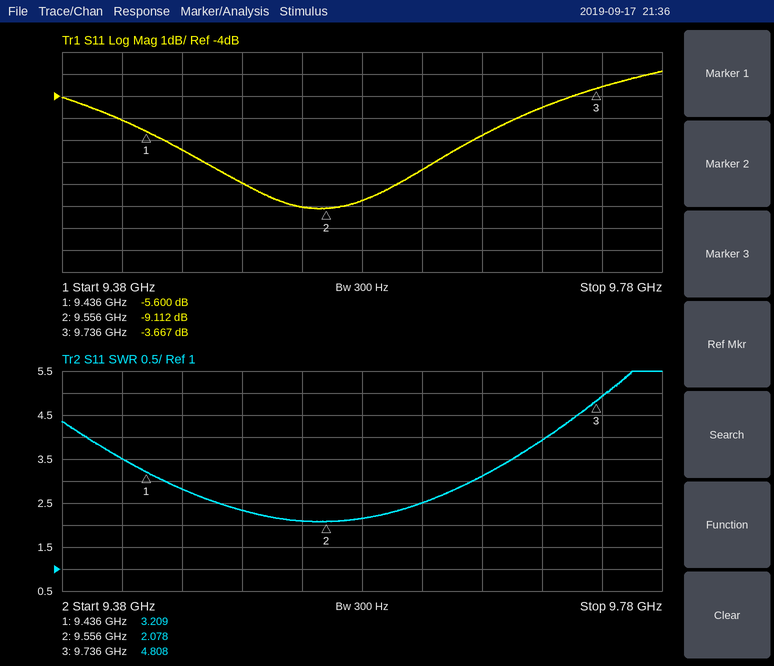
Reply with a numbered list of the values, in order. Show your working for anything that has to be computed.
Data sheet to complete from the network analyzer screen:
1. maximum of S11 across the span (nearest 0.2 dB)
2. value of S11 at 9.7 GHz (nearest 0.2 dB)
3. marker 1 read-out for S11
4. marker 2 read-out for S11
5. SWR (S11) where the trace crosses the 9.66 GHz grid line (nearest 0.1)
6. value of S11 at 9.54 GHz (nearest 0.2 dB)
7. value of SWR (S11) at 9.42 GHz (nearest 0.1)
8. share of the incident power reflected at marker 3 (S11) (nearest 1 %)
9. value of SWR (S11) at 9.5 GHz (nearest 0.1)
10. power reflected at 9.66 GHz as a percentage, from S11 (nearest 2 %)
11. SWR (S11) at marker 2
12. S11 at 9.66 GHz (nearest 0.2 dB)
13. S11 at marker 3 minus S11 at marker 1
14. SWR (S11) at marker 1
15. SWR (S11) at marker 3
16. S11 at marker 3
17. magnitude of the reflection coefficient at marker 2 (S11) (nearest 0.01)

1. -2.8 dB
2. -4.6 dB
3. -5.600 dB
4. -9.112 dB
5. 3.1
6. -9.0 dB
7. 3.5
8. 10^(-3.667/10) ≈ 43 %
9. 2.3
10. 10^(-5.8/10) ≈ 26 %
11. 2.078
12. -5.8 dB
13. -3.667 − (-5.6) = 1.933 dB
14. 3.209
15. 4.808
16. -3.667 dB
17. 10^(-9.112/20) ≈ 0.35
